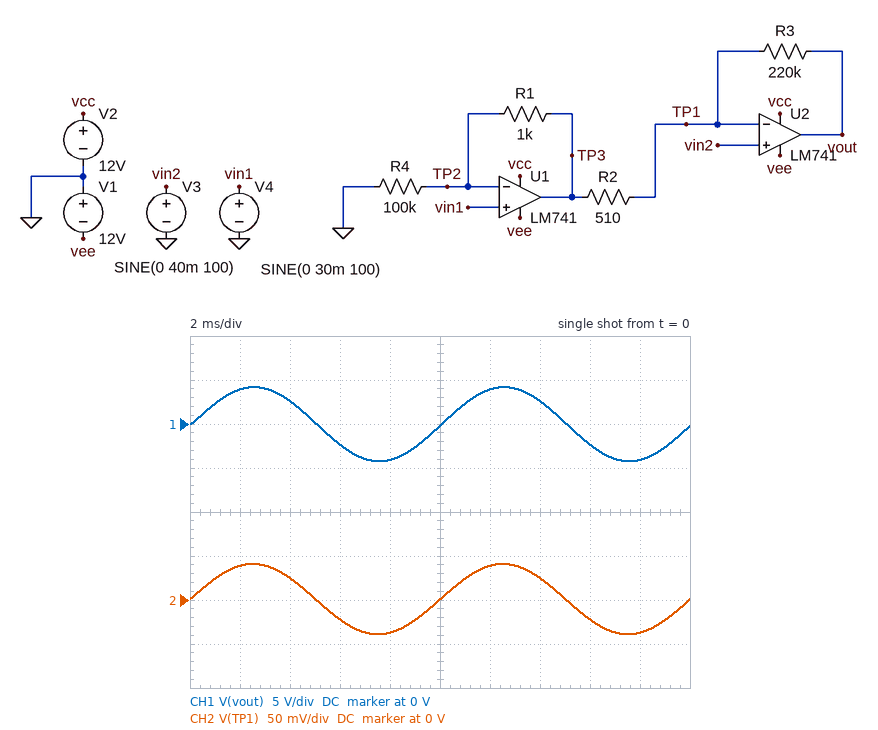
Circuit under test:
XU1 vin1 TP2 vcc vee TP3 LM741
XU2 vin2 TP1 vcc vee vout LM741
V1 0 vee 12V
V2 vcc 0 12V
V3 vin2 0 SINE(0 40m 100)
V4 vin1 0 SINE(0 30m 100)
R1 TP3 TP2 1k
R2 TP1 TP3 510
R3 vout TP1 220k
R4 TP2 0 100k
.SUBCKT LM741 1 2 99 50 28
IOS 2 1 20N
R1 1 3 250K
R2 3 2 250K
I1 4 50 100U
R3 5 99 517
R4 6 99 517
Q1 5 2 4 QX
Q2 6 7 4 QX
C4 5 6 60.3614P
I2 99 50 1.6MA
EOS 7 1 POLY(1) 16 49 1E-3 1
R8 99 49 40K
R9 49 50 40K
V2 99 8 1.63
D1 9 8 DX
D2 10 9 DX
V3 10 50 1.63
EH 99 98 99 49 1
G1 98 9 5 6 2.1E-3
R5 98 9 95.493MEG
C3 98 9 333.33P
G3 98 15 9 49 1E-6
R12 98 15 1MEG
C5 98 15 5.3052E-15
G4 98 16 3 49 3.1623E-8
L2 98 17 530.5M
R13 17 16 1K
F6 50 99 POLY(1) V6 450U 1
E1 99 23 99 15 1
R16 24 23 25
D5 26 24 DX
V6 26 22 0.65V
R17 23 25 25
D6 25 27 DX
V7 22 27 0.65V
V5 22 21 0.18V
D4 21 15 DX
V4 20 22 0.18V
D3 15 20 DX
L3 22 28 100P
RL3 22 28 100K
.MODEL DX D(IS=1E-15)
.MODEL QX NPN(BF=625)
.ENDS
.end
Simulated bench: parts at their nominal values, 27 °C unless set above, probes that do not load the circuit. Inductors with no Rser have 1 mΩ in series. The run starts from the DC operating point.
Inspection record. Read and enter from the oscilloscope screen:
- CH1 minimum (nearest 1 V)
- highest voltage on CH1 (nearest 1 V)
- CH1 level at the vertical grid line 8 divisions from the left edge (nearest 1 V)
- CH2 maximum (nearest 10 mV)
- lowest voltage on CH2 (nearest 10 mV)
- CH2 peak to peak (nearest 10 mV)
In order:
-4 V
4 V
-2 V
40 mV
-40 mV
80 mV
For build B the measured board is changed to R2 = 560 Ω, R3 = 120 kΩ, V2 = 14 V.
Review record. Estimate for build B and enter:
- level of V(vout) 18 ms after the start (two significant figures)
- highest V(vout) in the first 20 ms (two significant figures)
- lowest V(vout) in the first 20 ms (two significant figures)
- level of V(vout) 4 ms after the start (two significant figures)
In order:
-2.0 V
2.1 V
-2.1 V
1.3 V
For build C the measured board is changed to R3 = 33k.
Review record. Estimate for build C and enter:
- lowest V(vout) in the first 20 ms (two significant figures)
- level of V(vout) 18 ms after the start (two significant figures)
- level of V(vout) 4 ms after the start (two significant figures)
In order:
-670 mV
-640 mV
390 mV
